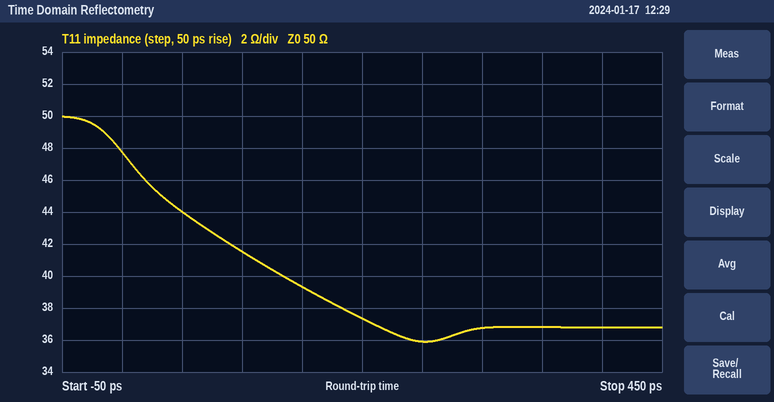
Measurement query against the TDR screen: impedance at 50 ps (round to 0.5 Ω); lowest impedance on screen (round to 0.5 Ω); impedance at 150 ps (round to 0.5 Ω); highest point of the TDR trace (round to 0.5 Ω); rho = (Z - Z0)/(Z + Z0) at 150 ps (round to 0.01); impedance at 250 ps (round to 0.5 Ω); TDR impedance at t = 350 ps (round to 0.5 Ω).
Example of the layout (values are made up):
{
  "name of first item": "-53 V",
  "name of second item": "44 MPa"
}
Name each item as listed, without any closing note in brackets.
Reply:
{
  "impedance at 50 ps": "44.0 Ω",
  "lowest impedance on screen": "36.0 Ω",
  "impedance at 150 ps": "39.5 Ω",
  "highest point of the TDR trace": "50.0 Ω",
  "rho = (Z - Z0)/(Z + Z0) at 150 ps": "-0.12",
  "impedance at 250 ps": "36.0 Ω",
  "TDR impedance at t = 350 ps": "37.0 Ω"
}
